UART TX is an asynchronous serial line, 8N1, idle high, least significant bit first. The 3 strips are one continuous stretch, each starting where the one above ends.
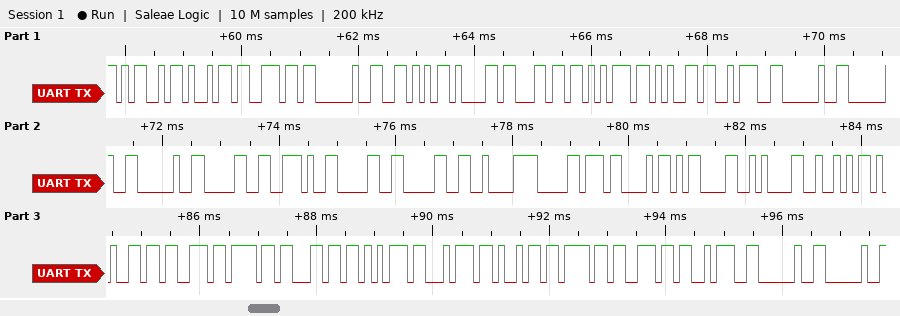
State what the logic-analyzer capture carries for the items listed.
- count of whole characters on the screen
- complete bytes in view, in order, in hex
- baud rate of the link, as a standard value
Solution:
35
4D 69 6E 20 56 61 6C 75 65 3A 20 20 20 30 2E 30 30 C2 B0 43 0D 0A 52 65 73 6F 6C 75 74 69 6F 6E 3A 20 20
9600 baud
